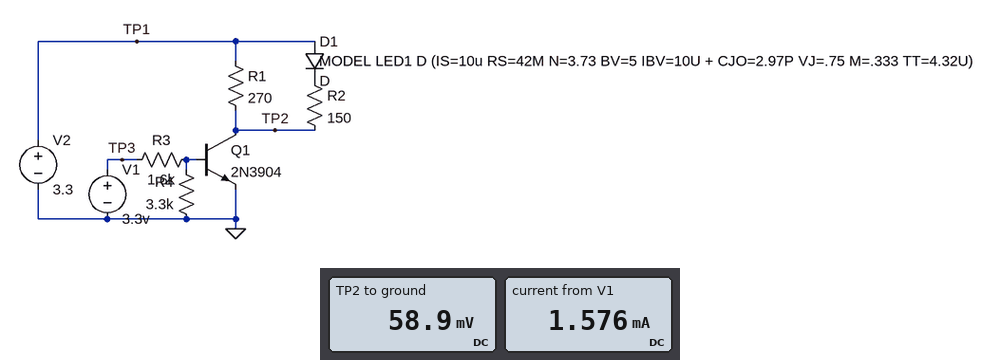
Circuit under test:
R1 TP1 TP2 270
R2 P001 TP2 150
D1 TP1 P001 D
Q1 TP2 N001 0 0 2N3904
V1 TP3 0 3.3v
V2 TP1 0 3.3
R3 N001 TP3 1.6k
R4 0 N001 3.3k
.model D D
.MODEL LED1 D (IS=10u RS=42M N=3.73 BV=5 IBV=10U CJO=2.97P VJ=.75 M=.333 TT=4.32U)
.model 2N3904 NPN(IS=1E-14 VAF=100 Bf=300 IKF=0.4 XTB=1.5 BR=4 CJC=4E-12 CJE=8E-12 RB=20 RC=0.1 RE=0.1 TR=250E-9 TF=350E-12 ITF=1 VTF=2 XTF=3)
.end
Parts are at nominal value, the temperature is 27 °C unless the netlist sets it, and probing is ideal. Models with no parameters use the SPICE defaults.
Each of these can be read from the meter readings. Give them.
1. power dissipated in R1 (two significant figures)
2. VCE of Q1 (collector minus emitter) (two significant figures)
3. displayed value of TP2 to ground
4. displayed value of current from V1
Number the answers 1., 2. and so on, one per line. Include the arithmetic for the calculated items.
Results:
1. (3.3 V - 58.9 mV)^2 / 270 Ω = 39 mW
2. 58.9 mV = 59 mV
3. 58.9 mV
4. 1.576 mA
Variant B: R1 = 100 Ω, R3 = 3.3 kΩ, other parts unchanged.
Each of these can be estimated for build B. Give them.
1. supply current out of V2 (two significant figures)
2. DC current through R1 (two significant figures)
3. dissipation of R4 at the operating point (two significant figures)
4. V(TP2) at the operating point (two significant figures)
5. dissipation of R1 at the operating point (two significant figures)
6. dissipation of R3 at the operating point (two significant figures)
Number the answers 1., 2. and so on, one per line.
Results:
1. 48 mA
2. 32 mA
3. 180 µW
4. 110 mV
5. 100 mW
6. 1.9 mW
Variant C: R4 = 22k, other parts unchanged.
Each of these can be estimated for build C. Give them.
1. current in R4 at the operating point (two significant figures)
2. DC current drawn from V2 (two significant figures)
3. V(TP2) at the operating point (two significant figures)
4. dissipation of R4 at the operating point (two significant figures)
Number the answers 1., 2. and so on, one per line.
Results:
1. 36 µA
2. 29 mA
3. 56 mV
4. 28 µW
